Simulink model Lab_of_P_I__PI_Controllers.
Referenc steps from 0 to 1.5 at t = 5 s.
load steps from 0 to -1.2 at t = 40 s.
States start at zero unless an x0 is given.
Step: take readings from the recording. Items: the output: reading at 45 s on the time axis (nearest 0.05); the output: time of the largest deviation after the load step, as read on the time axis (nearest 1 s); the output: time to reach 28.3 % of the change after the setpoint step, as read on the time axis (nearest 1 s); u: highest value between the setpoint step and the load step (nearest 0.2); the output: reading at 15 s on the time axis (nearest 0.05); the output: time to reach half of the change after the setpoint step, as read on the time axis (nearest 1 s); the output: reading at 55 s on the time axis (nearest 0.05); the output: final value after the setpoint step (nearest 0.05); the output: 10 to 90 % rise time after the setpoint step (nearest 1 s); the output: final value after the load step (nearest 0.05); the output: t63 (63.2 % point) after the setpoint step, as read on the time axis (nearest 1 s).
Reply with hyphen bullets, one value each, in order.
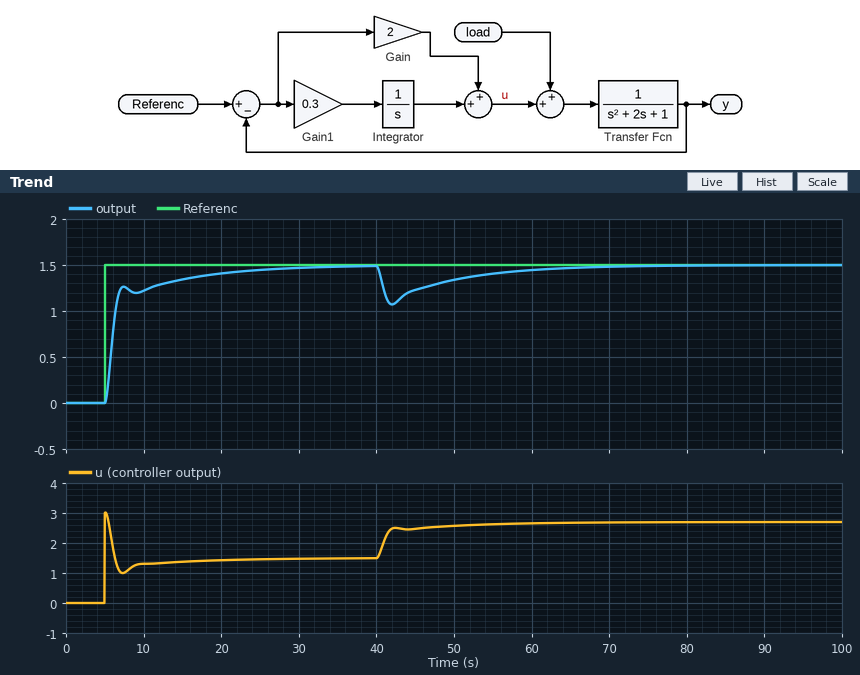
- 1.25
- 42 s
- 6 s
- 3.0
- 1.35
- 6 s
- 1.40
- 1.50
- 10 s
- 1.50
- 6 s
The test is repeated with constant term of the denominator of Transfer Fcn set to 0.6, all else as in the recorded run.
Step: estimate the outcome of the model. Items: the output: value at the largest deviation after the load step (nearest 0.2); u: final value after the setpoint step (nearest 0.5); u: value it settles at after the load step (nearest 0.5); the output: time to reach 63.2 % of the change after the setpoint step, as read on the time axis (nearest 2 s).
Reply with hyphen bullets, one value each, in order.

- 1.0
- 1.0
- 2.0
- 6 s
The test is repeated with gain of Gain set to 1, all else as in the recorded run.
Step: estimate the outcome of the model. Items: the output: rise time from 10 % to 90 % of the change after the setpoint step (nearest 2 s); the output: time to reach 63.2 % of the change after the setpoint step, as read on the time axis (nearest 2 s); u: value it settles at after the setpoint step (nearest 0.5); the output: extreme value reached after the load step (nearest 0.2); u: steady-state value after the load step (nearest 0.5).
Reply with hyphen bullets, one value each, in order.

- 8 s
- 8 s
- 1.5
- 1.0
- 2.5
